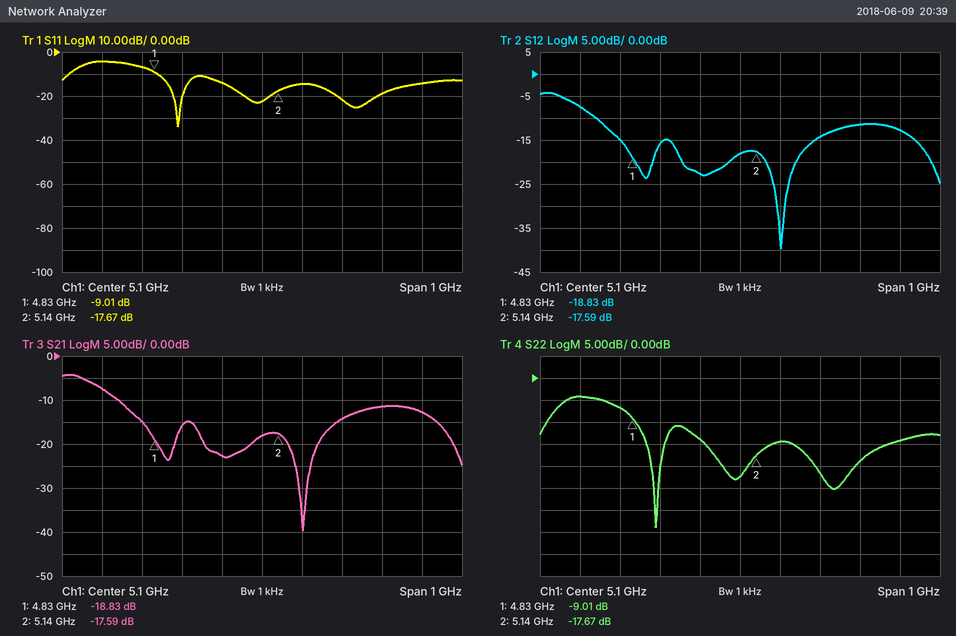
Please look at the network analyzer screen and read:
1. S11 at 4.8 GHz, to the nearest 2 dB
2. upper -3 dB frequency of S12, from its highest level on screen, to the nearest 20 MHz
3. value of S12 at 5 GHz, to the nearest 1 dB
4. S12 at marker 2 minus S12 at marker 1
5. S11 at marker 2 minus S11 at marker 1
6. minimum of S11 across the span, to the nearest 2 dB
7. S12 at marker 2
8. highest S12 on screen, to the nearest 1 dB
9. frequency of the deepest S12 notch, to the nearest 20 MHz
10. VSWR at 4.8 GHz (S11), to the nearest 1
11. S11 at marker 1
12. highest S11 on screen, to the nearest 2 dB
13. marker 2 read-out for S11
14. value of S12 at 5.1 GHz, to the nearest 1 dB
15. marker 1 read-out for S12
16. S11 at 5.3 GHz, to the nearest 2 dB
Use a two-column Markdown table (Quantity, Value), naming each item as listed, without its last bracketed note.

| Quantity | Value |
|---|---|
| S11 at 4.8 GHz, to the nearest 2 dB | -6 dB |
| upper -3 dB frequency of S12, from its highest level on screen, to the nearest 20 MHz | 4.70 GHz |
| value of S12 at 5 GHz, to the nearest 1 dB | -23 dB |
| S12 at marker 2 minus S12 at marker 1 | 1.24 dB |
| S11 at marker 2 minus S11 at marker 1 | -8.66 dB |
| minimum of S11 across the span, to the nearest 2 dB | -34 dB |
| S12 at marker 2 | -17.59 dB |
| highest S12 on screen, to the nearest 1 dB | -4 dB |
| frequency of the deepest S12 notch, to the nearest 20 MHz | 5.20 GHz |
| VSWR at 4.8 GHz (S11), to the nearest 1 | 3 |
| S11 at marker 1 | -9.01 dB |
| highest S11 on screen, to the nearest 2 dB | -4 dB |
| marker 2 read-out for S11 | -17.67 dB |
| value of S12 at 5.1 GHz, to the nearest 1 dB | -18 dB |
| marker 1 read-out for S12 | -18.83 dB |
| S11 at 5.3 GHz, to the nearest 2 dB | -22 dB |
